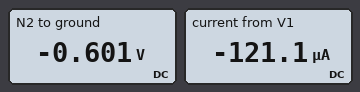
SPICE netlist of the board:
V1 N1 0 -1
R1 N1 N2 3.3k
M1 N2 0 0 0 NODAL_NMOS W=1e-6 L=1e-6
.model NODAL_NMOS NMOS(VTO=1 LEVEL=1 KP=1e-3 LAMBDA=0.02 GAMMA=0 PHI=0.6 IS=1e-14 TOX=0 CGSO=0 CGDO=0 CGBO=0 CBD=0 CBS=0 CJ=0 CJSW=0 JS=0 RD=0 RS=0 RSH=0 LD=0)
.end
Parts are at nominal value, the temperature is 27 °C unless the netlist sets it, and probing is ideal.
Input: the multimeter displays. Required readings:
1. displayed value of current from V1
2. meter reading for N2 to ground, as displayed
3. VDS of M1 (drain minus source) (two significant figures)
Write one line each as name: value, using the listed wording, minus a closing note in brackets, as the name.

displayed value of current from V1: -121.1 µA
meter reading for N2 to ground, as displayed: -0.601 V
VDS of M1 (drain minus source): -600 mV
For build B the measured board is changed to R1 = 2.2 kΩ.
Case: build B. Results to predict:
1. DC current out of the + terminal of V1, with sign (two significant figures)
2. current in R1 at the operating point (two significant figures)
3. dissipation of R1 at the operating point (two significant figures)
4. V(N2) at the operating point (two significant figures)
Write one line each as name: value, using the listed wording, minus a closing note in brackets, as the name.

DC current out of the + terminal of V1, with sign: -180 µA
current in R1 at the operating point: 180 µA
dissipation of R1 at the operating point: 69 µW
V(N2) at the operating point: -610 mV
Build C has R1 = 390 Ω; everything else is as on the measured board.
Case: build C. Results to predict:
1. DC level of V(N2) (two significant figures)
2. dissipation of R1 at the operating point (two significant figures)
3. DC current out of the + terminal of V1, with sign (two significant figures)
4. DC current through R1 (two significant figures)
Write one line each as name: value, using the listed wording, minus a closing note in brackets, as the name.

DC level of V(N2): -650 mV
dissipation of R1 at the operating point: 310 µW
DC current out of the + terminal of V1, with sign: -890 µA
DC current through R1: 890 µA
